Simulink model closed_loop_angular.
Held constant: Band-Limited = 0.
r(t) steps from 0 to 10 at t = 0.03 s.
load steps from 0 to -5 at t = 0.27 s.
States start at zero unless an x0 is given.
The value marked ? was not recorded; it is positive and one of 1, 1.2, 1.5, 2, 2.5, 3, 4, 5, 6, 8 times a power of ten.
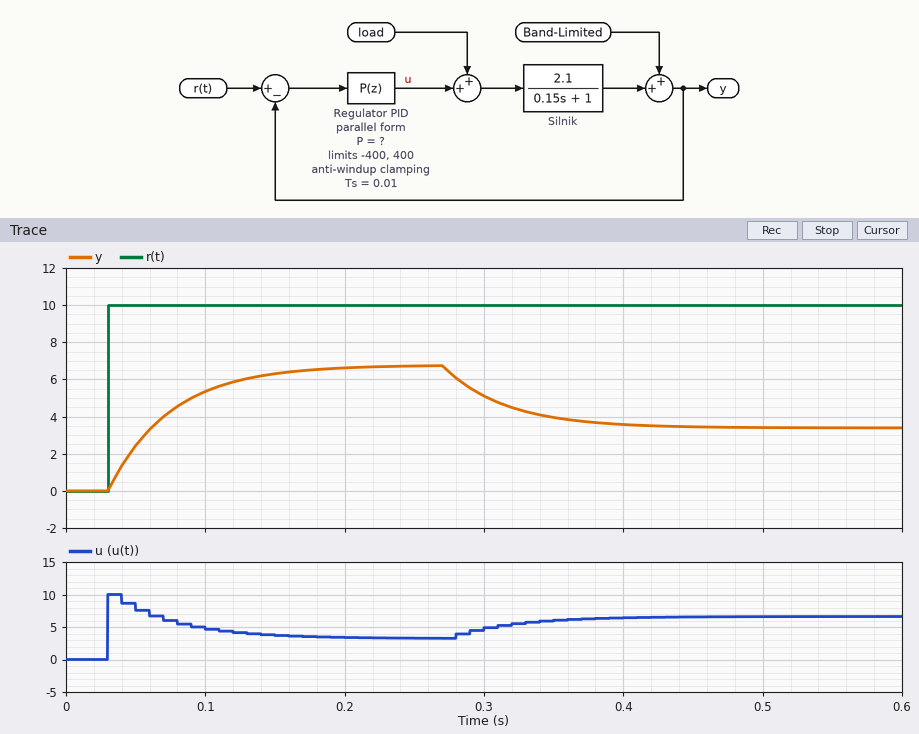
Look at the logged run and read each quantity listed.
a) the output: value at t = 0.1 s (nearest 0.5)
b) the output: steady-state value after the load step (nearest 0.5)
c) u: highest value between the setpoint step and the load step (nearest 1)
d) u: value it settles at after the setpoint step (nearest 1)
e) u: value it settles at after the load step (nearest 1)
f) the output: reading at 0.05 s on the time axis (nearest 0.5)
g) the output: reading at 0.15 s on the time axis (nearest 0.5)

5.5
3.5
10
3
7
2.5
6.5
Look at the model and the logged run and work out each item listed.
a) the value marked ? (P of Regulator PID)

1
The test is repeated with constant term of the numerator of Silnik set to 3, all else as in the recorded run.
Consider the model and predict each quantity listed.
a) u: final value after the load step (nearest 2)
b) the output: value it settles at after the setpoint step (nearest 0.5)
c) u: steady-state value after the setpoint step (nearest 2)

6
7.5
2
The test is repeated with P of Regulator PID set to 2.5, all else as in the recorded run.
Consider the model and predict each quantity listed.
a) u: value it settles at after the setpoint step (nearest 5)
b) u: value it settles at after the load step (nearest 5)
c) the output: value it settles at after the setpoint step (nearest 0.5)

5
10
8.5
